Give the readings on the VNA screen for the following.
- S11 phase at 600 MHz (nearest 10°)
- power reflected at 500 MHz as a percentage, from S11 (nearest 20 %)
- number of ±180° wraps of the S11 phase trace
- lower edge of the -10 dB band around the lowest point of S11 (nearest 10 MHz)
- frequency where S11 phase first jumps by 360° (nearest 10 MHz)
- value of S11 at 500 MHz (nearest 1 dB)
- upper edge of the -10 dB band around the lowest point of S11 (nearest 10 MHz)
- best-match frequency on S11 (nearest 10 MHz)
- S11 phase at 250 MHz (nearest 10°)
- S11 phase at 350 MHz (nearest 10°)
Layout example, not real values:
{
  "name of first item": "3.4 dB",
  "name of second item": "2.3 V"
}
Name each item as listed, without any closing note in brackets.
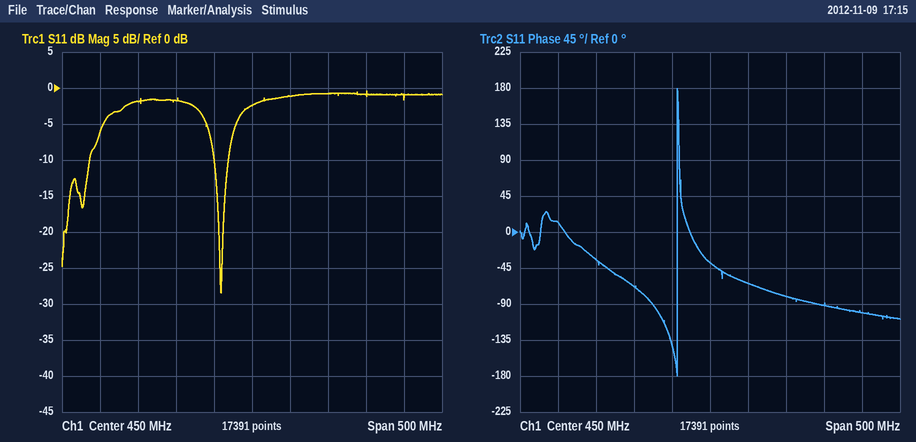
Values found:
{
  "S11 phase at 600 MHz": "-90°",
  "power reflected at 500 MHz as a percentage, from S11": "80 %",
  "number of ±180° wraps of the S11 phase trace": "1",
  "lower edge of the -10 dB band around the lowest point of S11": "400 MHz",
  "frequency where S11 phase first jumps by 360°": "410 MHz",
  "value of S11 at 500 MHz": "-1 dB",
  "upper edge of the -10 dB band around the lowest point of S11": "420 MHz",
  "best-match frequency on S11": "410 MHz",
  "S11 phase at 250 MHz": "10°",
  "S11 phase at 350 MHz": "-70°"
}
